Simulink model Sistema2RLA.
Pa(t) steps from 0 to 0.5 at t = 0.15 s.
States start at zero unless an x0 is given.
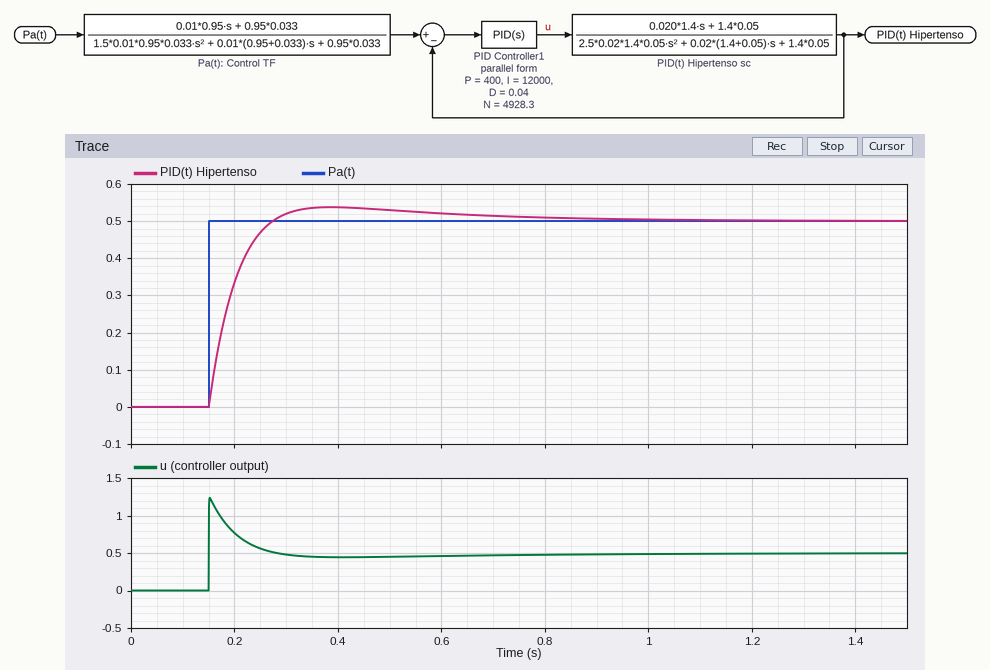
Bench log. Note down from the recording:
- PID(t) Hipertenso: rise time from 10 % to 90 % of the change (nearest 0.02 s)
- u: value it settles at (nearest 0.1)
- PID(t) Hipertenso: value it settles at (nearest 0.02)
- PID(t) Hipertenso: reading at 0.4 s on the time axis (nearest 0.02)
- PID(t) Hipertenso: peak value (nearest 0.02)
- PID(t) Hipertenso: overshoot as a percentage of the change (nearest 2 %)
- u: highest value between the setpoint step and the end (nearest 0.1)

0.08 s
0.5
0.50
0.54
0.54
8 %
1.2
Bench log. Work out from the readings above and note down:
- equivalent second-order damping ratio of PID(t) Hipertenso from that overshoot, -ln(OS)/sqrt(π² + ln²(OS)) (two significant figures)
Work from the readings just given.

0.63
